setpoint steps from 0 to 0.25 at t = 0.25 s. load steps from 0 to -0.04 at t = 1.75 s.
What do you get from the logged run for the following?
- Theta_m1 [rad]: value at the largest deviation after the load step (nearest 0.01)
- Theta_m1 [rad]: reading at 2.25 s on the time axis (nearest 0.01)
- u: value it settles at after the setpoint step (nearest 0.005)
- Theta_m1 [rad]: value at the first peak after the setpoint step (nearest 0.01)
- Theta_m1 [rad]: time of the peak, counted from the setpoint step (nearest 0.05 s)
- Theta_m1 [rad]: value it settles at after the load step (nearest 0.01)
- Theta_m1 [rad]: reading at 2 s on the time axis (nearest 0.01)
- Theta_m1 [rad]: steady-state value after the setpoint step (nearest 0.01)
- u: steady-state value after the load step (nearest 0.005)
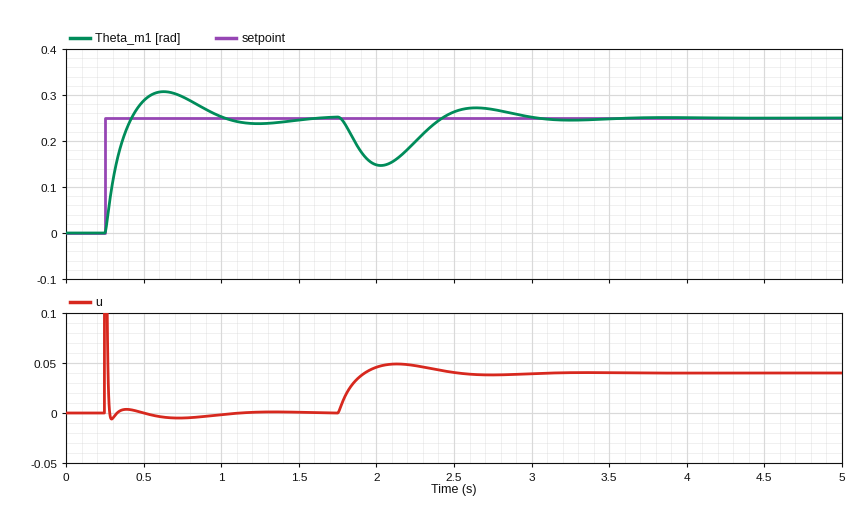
0.15
0.20
0.000
0.31
0.40 s
0.25
0.15
0.25
0.040
